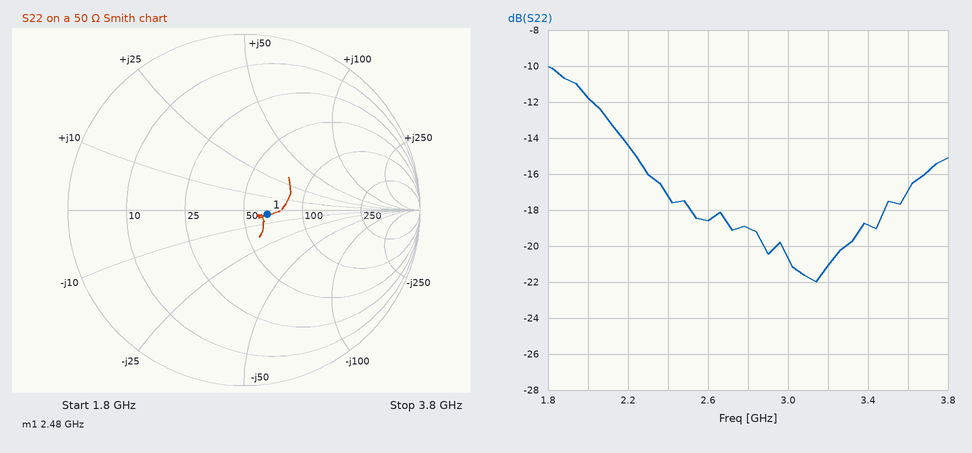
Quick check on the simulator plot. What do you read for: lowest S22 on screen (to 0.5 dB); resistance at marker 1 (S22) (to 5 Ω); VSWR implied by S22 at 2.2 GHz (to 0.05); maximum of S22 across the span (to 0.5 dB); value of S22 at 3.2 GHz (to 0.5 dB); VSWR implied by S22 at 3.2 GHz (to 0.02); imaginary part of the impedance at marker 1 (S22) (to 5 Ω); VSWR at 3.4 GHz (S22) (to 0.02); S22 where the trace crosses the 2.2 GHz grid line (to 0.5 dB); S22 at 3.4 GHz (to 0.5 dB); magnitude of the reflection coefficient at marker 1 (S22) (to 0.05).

-22.0 dB
65 Ω
1.45
-10.0 dB
-21.0 dB
1.20
-5 Ω
1.26
-14.5 dB
-19.0 dB
0.15
